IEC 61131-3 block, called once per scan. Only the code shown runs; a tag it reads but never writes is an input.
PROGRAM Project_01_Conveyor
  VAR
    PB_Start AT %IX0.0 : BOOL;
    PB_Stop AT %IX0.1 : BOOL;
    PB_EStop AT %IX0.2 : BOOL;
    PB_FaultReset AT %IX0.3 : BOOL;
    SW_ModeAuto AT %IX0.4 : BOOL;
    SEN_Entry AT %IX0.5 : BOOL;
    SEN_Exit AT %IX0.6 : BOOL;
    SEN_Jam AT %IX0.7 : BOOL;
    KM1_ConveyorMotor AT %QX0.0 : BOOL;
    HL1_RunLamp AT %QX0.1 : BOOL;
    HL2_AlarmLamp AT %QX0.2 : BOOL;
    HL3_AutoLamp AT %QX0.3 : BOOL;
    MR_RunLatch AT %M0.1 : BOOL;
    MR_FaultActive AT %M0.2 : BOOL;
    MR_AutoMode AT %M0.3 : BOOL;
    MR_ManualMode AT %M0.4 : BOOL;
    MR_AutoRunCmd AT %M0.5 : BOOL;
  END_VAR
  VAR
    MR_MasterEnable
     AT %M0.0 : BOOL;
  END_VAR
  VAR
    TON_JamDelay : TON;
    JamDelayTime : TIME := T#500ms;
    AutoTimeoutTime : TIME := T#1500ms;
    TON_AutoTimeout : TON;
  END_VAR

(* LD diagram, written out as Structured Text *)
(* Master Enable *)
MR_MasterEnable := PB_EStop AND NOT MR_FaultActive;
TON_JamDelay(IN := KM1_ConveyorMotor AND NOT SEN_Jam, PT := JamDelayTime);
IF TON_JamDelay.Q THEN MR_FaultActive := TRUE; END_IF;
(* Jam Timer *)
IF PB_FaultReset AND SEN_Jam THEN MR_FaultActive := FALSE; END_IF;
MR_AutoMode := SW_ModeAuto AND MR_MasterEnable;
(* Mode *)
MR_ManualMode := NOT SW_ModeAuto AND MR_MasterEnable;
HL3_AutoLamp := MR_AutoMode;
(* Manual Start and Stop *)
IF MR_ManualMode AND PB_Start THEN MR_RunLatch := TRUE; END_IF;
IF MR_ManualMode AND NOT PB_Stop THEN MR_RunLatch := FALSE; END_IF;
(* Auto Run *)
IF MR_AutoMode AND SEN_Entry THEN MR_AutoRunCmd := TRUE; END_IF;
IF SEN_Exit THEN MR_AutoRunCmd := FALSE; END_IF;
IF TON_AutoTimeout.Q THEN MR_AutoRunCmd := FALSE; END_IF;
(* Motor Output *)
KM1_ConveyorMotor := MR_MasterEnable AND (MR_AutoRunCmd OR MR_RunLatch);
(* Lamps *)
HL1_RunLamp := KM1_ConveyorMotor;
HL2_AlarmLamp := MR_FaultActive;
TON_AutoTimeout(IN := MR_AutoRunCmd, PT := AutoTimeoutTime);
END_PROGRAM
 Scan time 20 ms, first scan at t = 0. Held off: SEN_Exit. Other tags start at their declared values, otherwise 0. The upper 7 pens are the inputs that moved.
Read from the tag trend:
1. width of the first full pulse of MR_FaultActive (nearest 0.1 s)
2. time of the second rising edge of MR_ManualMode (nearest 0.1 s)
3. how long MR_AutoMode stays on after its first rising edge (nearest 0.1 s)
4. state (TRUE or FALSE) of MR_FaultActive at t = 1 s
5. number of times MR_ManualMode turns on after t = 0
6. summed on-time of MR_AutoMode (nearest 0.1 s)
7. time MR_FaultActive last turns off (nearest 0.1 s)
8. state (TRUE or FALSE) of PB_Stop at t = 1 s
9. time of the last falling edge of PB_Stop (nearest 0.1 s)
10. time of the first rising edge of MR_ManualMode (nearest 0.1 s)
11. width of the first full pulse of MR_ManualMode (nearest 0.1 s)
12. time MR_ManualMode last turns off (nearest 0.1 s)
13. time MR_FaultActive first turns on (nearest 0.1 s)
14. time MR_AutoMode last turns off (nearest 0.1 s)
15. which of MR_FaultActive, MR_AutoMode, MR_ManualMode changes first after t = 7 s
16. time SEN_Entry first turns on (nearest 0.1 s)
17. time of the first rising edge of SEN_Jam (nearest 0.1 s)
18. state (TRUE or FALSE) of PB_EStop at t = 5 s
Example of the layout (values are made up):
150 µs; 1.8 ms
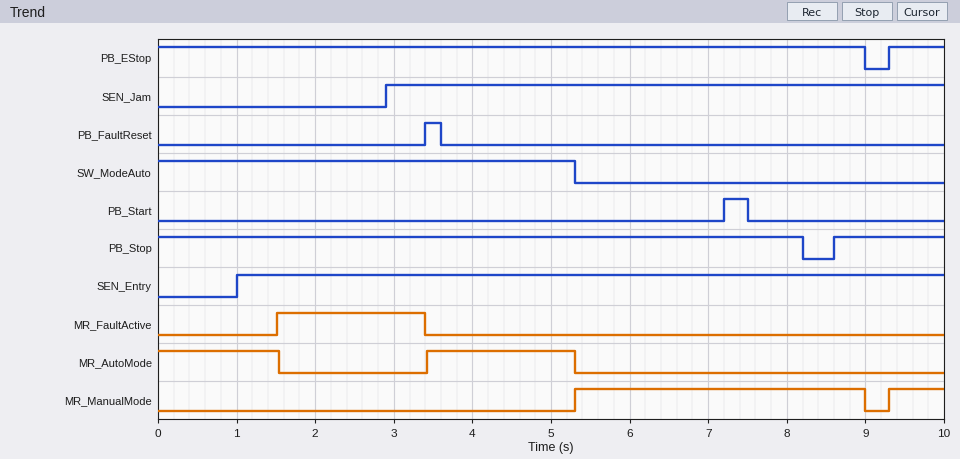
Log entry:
1.9 s; 9.3 s; 1.9 s; FALSE; 2; 3.4 s; 3.4 s; TRUE; 8.2 s; 5.3 s; 3.7 s; 9.0 s; 1.5 s; 5.3 s; MR_ManualMode; 1.0 s; 2.9 s; TRUE
